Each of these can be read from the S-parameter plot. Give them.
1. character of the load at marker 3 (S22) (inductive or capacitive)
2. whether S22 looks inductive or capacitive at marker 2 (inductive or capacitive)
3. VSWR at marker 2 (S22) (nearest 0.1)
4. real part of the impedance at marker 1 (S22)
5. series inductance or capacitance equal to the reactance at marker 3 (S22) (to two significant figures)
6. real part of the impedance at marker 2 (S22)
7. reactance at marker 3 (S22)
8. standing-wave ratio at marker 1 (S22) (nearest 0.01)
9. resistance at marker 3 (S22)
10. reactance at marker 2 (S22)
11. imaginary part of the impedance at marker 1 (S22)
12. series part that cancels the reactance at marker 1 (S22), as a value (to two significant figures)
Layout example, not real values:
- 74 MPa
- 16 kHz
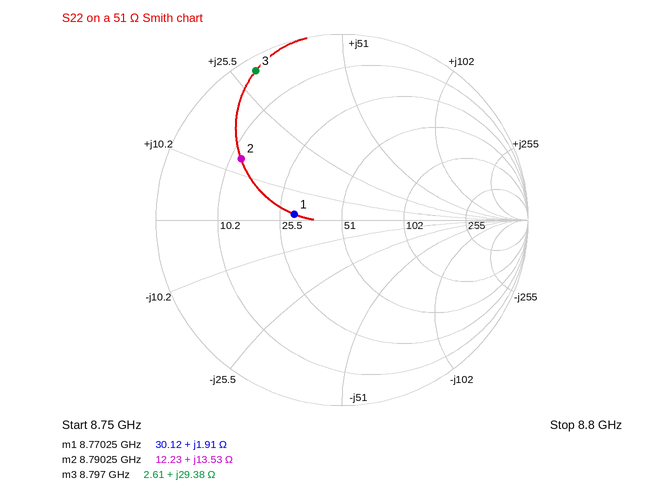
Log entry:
- inductive
- inductive
- 4.5
- 30.12 Ω
- 530 pH
- 12.23 Ω
- +29.38 Ω
- 1.70
- 2.61 Ω
- +13.53 Ω
- +1.91 Ω
- 9.5 pF
